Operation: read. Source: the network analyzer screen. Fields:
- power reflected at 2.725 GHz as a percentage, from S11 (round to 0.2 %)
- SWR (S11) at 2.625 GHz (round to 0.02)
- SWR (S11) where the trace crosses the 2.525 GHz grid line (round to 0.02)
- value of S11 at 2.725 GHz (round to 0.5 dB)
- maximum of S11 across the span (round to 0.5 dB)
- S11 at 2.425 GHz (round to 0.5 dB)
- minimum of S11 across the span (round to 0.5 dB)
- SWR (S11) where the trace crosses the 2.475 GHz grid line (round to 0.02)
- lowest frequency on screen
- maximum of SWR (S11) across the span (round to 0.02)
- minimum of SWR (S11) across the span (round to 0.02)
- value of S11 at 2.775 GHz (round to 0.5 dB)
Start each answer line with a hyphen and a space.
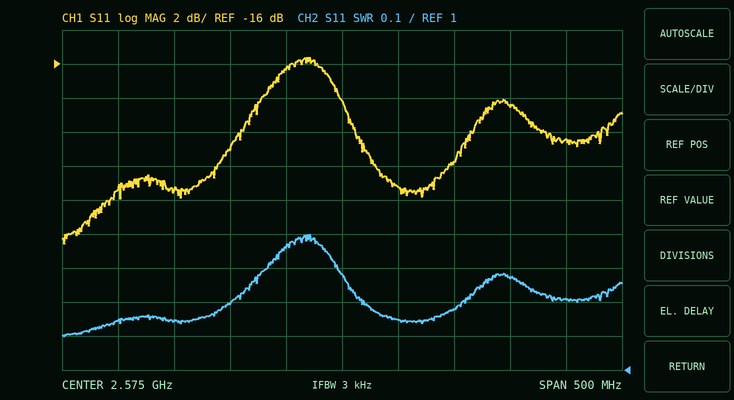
- 1.4 %
- 1.14
- 1.36
- -18.5 dB
- -15.5 dB
- -23.5 dB
- -26.5 dB
- 1.20
- 2.325 GHz
- 1.40
- 1.10
- -20.5 dB
